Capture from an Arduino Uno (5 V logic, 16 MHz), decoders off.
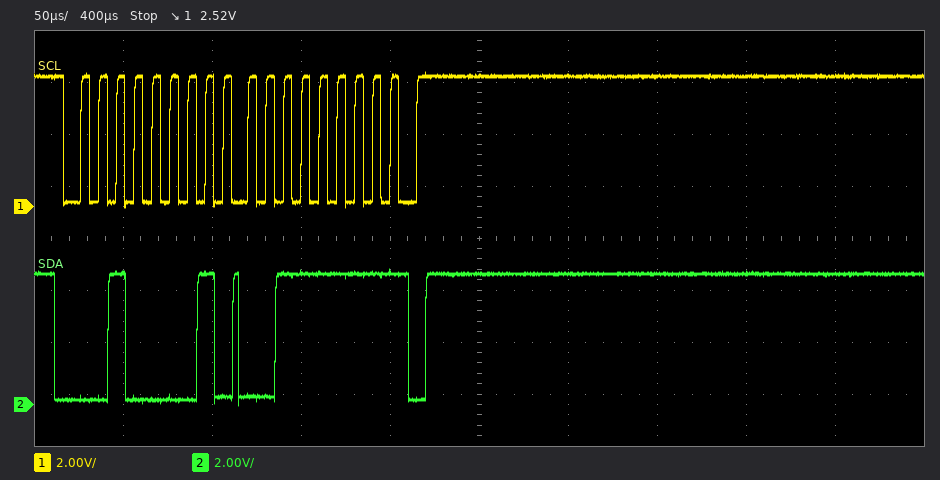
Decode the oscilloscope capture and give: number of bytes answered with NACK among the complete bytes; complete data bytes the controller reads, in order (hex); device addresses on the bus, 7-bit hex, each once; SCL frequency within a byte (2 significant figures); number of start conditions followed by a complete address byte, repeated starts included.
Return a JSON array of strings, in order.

["1", "3F", "0x10", "100 kHz", "1"]
